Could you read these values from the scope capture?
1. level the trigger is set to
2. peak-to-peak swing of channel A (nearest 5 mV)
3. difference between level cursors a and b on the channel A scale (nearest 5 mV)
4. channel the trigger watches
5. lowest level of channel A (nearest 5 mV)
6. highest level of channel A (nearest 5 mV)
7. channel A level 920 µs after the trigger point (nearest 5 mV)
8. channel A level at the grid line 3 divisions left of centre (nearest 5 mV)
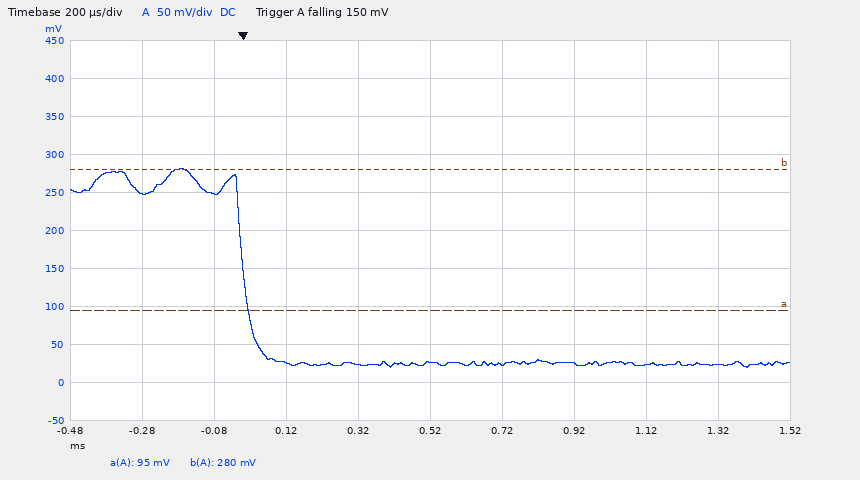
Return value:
150 mV
260 mV
185 mV
channel A
20 mV
280 mV
25 mV
250 mV
